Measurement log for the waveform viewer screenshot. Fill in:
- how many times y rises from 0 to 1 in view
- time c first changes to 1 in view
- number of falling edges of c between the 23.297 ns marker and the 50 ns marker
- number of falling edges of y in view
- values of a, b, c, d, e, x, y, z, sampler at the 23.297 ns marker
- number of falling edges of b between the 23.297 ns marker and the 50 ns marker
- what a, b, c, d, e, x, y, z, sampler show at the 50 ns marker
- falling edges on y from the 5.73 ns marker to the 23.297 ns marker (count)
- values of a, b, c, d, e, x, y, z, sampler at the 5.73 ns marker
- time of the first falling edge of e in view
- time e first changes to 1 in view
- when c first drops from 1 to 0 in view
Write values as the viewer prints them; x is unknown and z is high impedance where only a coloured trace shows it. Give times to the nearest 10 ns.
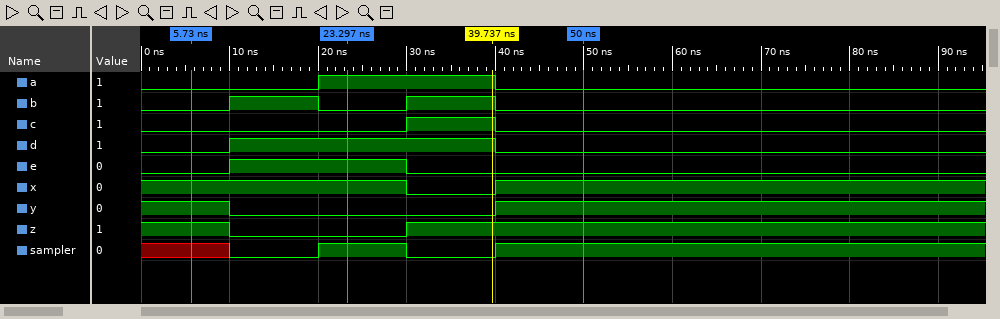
1
30 ns
1
1
a=1, b=0, c=0, d=1, e=1, x=1, y=0, z=0, sampler=1
1
a=0, b=0, c=0, d=0, e=0, x=1, y=1, z=1, sampler=1
1
a=0, b=0, c=0, d=0, e=0, x=1, y=1, z=1, sampler=x
30 ns
10 ns
40 ns
